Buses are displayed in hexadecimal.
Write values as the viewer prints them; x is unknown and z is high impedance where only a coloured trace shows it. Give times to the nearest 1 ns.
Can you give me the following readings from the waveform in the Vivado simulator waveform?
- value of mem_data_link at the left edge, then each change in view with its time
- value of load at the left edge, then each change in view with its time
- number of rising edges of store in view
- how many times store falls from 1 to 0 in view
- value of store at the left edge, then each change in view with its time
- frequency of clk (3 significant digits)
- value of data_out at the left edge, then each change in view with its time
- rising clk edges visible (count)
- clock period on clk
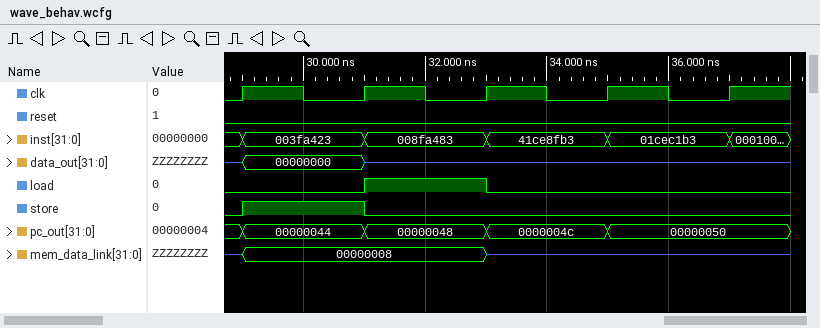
z, 00000008 at 29 ns, z at 33 ns
0, 1 at 31 ns, 0 at 33 ns
1
1
0, 1 at 29 ns, 0 at 31 ns
500 MHz
z, 00000000 at 29 ns, z at 31 ns
5
2 ns
